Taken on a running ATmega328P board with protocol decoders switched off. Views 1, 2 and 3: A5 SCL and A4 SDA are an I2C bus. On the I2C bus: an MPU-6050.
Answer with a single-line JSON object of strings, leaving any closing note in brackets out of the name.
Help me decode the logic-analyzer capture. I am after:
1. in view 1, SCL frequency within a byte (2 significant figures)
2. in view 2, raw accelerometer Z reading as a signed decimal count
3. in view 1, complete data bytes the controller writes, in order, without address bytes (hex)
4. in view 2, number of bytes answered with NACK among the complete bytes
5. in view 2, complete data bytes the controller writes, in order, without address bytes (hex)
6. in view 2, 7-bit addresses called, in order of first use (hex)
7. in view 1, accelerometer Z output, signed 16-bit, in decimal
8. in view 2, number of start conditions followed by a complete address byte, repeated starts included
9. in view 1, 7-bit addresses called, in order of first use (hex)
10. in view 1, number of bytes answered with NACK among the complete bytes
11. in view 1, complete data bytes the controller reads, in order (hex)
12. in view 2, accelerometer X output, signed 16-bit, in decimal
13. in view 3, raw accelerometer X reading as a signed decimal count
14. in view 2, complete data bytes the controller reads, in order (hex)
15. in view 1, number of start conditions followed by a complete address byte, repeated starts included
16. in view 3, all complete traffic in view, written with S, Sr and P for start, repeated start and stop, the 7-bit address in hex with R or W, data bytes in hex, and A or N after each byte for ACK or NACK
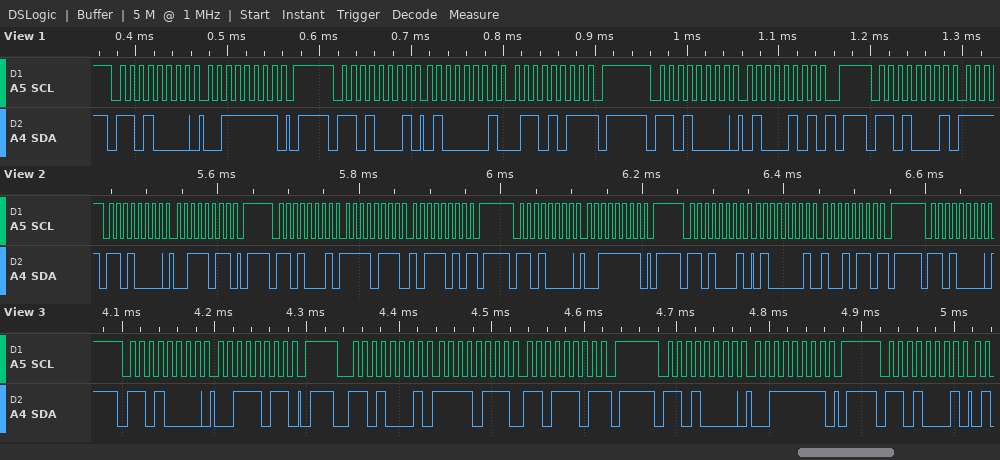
{"in view 1, SCL frequency within a byte": "100 kHz", "in view 2, raw accelerometer Z reading as a signed decimal count": "16790", "in view 1, complete data bytes the controller writes, in order, without address bytes": "3F 45", "in view 2, number of bytes answered with NACK among the complete bytes": "2", "in view 2, complete data bytes the controller writes, in order, without address bytes": "3B 3F", "in view 2, 7-bit addresses called, in order of first use": "0x68", "in view 1, accelerometer Z output, signed 16-bit, in decimal": "16747", "in view 2, number of start conditions followed by a complete address byte, repeated starts included": "5", "in view 1, 7-bit addresses called, in order of first use": "0x68", "in view 1, number of bytes answered with NACK among the complete bytes": "1", "in view 1, complete data bytes the controller reads, in order": "41 6B", "in view 2, accelerometer X output, signed 16-bit, in decimal": "-2118", "in view 3, raw accelerometer X reading as a signed decimal count": "-2083", "in view 2, complete data bytes the controller reads, in order": "F7 BA 41 96", "in view 1, number of start conditions followed by a complete address byte, repeated starts included": "4", "in view 3, all complete traffic in view, written with S, Sr and P for start, repeated start and stop, the 7-bit address in hex with R or W, data bytes in hex, and A or N after each byte for ACK or NACK": "S 68W A 3B A P S 68R A F7 A DD N P S 68W A 3F A P S 68R A"}
